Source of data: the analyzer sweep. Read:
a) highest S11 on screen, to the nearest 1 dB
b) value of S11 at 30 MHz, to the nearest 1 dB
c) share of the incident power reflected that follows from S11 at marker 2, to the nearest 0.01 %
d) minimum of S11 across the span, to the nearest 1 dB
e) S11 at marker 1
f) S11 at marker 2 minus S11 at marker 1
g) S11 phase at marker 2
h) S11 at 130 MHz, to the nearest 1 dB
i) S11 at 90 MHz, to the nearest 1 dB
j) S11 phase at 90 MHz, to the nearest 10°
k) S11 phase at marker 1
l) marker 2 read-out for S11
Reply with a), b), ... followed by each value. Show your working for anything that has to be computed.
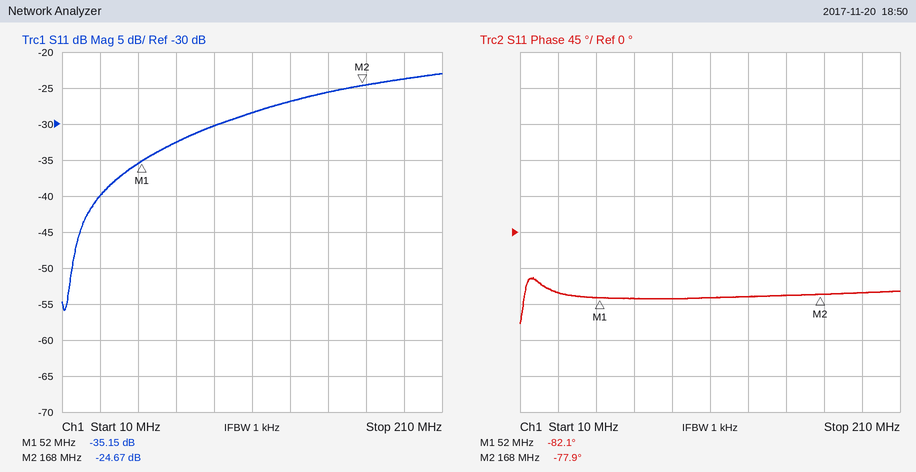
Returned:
a) -23 dB
b) -40 dB
c) 10^(-24.67/10) ≈ 0.34 %
d) -56 dB
e) -35.15 dB
f) -24.67 − (-35.15) = 10.48 dB
g) -77.9°
h) -27 dB
i) -30 dB
j) -80°
k) -82.1°
l) -24.67 dB
